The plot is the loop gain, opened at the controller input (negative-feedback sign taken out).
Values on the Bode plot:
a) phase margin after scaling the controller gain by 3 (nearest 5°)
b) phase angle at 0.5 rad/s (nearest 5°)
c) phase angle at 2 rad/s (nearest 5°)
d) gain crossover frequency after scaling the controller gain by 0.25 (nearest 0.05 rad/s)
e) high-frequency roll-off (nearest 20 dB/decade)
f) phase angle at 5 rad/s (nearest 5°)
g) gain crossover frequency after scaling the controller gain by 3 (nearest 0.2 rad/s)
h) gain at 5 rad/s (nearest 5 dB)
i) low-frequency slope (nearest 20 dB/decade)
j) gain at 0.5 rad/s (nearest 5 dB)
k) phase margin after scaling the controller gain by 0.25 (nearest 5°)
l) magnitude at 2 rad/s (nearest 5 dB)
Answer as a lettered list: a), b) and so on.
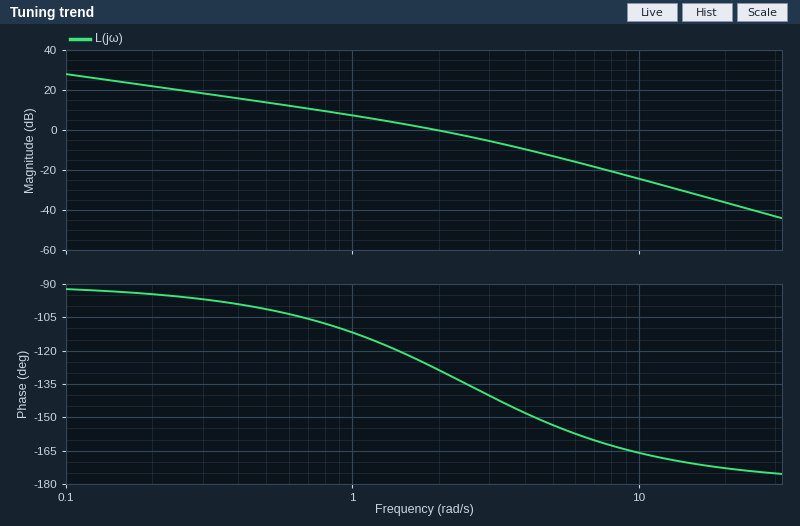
a) 30°
b) -100°
c) -130°
d) 0.60 rad/s
e) -40 dB/decade
f) -155°
g) 4.0 rad/s
h) -15 dB
i) -20 dB/decade
j) 15 dB
k) 75°
l) 0 dB
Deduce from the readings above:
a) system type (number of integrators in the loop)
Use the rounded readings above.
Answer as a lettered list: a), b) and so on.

a) 1
